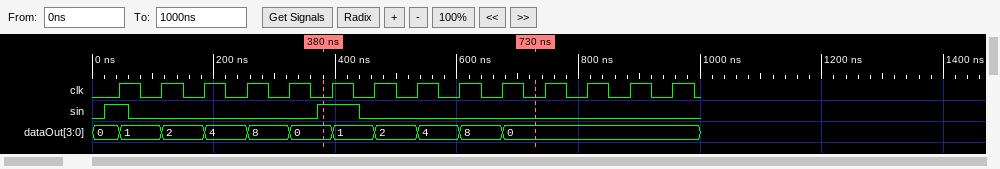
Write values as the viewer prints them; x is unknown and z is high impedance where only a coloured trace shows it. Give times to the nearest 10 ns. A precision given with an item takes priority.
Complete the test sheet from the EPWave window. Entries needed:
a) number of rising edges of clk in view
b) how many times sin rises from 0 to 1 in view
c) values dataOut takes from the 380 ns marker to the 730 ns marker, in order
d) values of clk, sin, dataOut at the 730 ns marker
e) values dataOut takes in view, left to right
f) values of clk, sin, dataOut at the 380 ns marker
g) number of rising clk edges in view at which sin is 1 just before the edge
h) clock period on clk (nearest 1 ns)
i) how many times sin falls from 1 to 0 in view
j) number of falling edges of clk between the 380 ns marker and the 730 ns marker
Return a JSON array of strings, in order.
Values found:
["14", "2", "0, 1, 2, 4, 8, 0", "clk=0, sin=0, dataOut=0", "0, 1, 2, 4, 8, 0, 1, 2, 4, 8, 0", "clk=0, sin=1, dataOut=0", "2", "70 ns", "2", "5"]
